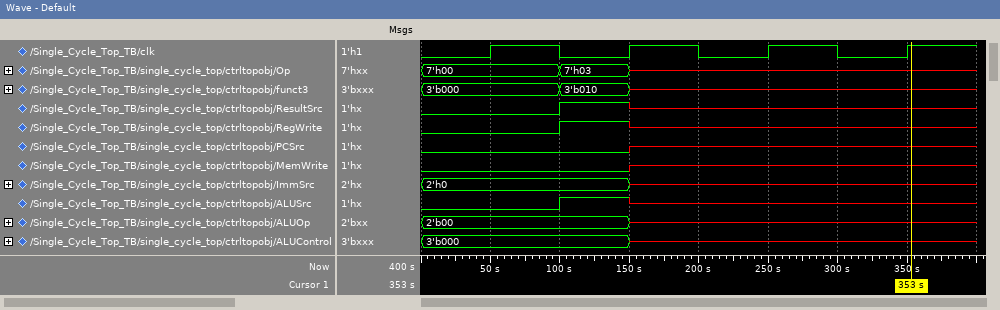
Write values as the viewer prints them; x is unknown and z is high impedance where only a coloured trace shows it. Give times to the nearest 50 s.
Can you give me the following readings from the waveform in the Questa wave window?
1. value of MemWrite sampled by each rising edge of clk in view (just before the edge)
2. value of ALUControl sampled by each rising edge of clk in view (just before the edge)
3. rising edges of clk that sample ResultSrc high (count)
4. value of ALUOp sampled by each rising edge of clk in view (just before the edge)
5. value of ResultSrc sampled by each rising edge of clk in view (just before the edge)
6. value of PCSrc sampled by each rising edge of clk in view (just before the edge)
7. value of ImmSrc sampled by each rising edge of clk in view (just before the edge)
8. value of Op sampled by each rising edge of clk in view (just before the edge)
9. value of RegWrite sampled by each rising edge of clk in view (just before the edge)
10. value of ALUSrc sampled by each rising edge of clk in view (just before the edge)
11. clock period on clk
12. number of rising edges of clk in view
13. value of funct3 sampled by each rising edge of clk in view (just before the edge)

0 0 x x
3'b000, 3'b000, x, x
1
2'b00, 2'b00, x, x
0 1 x x
0 0 x x
2'h0, 2'h0, x, x
7'h00, 7'h03, x, x
0 1 x x
0 1 x x
100 s
4
3'b000, 3'b010, x, x
